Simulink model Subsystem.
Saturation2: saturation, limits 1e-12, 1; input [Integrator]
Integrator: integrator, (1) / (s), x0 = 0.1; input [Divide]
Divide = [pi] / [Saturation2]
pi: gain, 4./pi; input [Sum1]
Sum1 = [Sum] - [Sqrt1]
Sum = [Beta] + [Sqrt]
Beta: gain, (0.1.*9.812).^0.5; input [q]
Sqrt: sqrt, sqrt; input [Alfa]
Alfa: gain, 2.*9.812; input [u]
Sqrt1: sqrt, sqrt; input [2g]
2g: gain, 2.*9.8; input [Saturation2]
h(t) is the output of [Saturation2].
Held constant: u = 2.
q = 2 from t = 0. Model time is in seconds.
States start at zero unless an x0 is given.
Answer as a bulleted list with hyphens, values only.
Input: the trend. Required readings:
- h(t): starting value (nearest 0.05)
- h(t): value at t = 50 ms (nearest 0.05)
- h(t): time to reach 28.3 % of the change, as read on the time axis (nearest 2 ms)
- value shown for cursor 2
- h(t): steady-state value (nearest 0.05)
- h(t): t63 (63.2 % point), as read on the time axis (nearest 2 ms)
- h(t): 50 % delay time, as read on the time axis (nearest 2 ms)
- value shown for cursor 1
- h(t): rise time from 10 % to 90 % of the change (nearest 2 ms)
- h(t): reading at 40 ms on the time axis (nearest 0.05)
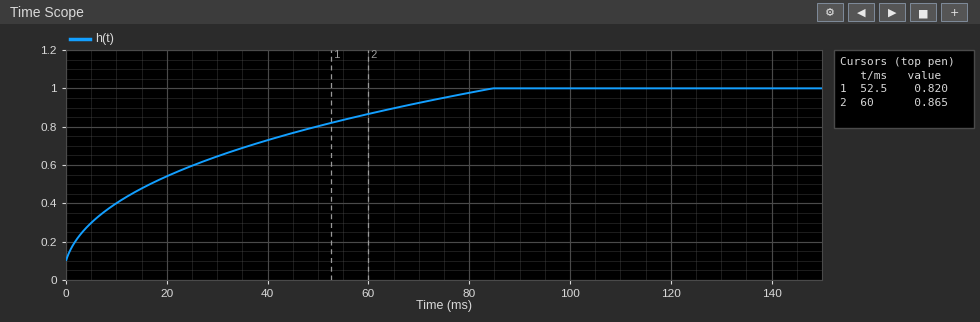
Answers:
- 0.10
- 0.80
- 8 ms
- 0.865
- 1.00
- 32 ms
- 20 ms
- 0.820
- 66 ms
- 0.75
